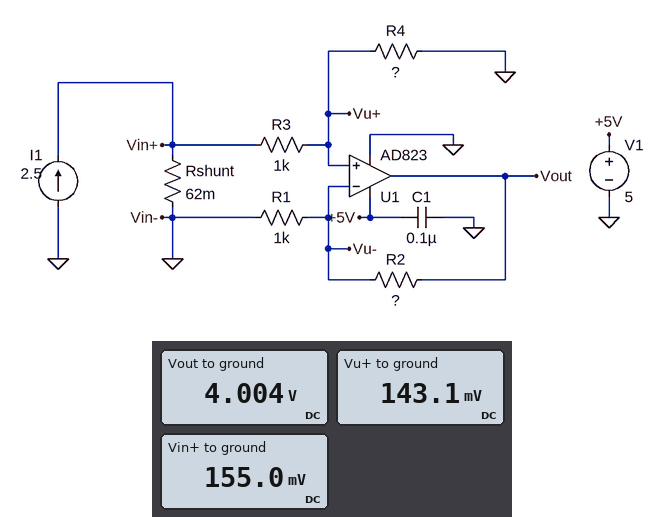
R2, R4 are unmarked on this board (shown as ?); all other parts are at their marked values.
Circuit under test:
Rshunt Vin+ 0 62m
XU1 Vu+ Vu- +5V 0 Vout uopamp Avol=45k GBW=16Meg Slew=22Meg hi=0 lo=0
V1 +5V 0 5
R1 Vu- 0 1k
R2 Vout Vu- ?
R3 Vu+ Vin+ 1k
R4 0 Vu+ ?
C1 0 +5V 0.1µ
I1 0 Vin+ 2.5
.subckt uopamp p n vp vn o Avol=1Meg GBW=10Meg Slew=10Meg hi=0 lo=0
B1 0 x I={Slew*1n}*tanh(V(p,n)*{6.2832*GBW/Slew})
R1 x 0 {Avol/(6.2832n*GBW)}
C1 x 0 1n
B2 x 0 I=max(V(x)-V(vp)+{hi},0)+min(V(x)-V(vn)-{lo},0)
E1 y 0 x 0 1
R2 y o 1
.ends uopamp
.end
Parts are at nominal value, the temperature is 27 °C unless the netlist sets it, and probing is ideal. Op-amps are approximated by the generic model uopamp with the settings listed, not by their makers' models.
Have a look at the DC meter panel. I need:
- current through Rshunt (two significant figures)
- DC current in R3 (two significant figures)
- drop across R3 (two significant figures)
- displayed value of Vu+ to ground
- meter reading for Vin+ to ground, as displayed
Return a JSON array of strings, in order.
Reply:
["2.5 A", "12 µA", "12 mV", "143.1 mV", "155.0 mV"]
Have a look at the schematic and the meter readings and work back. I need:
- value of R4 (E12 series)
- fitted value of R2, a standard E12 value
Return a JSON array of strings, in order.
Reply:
["12 kΩ", "27 kΩ"]
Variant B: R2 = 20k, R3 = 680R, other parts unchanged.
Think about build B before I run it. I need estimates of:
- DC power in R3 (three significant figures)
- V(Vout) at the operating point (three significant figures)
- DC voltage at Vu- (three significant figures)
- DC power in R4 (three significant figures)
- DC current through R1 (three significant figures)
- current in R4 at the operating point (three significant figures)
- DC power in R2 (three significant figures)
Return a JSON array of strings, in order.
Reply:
["102 nW", "3.08 V", "147 mV", "1.79 µW", "147 µA", "12.2 µA", "430 µW"]
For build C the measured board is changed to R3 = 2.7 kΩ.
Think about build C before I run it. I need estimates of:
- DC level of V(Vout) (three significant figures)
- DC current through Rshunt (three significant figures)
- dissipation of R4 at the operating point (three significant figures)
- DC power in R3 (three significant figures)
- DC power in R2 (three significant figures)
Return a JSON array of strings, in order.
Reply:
["3.54 V", "2.50 A", "1.33 µW", "300 nW", "432 µW"]
